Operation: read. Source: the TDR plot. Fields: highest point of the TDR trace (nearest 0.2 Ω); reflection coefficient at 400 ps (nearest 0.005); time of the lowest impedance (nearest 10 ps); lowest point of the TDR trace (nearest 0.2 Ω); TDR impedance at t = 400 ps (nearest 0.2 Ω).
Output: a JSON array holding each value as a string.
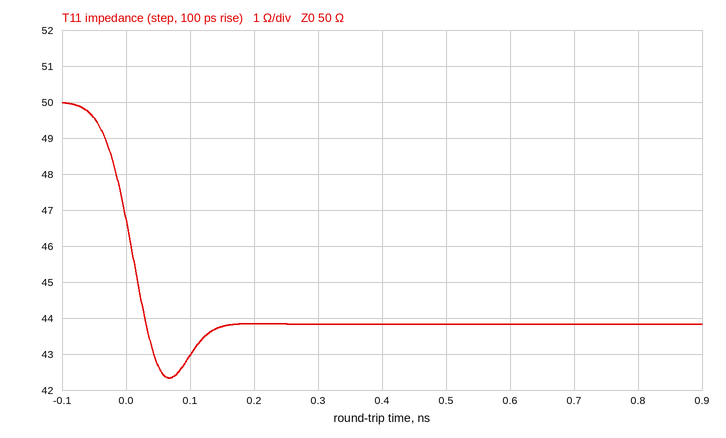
["50.0 Ω", "-0.065", "70 ps", "42.4 Ω", "43.8 Ω"]
